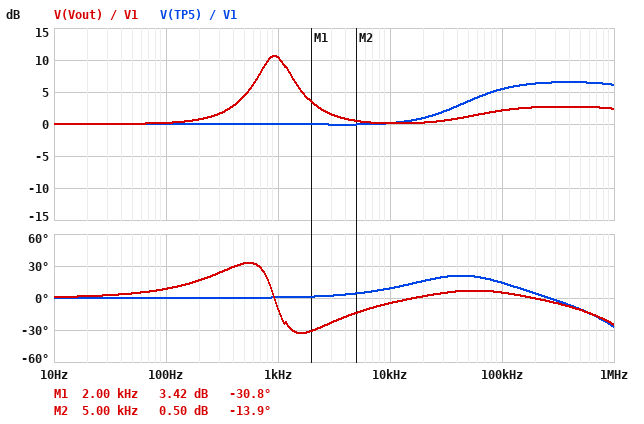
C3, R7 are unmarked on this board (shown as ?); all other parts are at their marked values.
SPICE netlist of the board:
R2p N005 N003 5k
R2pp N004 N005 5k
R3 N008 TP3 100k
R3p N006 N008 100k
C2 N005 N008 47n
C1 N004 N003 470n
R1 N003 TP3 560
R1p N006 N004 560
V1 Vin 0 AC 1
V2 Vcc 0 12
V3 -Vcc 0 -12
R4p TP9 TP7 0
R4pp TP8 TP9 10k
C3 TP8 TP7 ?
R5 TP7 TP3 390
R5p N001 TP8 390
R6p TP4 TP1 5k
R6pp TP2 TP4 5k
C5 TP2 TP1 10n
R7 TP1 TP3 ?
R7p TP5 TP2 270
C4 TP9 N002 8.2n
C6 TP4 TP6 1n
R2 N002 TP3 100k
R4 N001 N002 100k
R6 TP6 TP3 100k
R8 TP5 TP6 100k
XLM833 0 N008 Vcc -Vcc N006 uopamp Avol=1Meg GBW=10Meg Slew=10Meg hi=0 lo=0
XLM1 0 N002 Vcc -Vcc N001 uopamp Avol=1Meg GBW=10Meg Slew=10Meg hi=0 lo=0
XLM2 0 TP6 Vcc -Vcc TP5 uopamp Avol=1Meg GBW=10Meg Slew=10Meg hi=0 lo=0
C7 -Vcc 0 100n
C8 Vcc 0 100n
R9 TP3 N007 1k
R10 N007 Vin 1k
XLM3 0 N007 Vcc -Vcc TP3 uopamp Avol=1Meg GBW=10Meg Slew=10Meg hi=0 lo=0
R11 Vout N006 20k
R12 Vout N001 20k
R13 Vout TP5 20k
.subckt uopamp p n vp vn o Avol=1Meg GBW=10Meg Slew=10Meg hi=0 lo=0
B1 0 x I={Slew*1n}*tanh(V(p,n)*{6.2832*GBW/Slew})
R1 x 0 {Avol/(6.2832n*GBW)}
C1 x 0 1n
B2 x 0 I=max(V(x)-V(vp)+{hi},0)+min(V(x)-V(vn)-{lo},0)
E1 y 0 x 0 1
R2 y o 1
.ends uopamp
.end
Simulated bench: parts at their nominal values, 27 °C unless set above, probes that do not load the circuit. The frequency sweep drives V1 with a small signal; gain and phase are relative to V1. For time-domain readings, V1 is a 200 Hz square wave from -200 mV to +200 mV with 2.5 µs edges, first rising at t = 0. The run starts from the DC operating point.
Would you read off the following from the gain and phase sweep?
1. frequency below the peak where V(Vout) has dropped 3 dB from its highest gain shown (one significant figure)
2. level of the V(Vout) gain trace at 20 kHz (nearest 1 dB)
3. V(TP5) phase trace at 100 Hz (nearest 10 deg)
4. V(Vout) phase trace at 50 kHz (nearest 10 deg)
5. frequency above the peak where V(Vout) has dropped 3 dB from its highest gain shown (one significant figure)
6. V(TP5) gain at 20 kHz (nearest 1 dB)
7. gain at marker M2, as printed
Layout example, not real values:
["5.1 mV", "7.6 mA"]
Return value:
["700 Hz", "0 dB", "0 deg", "10 deg", "1 kHz", "1 dB", "0.50 dB"]
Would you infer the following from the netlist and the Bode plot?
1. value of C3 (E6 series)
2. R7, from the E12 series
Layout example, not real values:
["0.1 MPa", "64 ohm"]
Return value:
["100 nF", "120 Ω"]
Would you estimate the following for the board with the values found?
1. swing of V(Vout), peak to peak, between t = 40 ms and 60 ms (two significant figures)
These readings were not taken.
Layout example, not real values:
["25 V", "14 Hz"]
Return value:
["1.2 V"]
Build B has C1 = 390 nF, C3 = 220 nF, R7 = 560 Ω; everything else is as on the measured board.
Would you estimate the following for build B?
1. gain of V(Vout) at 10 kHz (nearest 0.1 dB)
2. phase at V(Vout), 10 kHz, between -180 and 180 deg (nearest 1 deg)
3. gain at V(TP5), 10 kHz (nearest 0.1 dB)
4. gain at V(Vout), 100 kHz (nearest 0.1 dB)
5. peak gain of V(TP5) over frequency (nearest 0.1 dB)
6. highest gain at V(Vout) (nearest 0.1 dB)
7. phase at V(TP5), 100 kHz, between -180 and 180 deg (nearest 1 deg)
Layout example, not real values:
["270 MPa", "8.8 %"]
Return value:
["-0.2 dB", "-9 deg", "-0.7 dB", "-1.5 dB", "0.1 dB", "7.2 dB", "-11 deg"]
